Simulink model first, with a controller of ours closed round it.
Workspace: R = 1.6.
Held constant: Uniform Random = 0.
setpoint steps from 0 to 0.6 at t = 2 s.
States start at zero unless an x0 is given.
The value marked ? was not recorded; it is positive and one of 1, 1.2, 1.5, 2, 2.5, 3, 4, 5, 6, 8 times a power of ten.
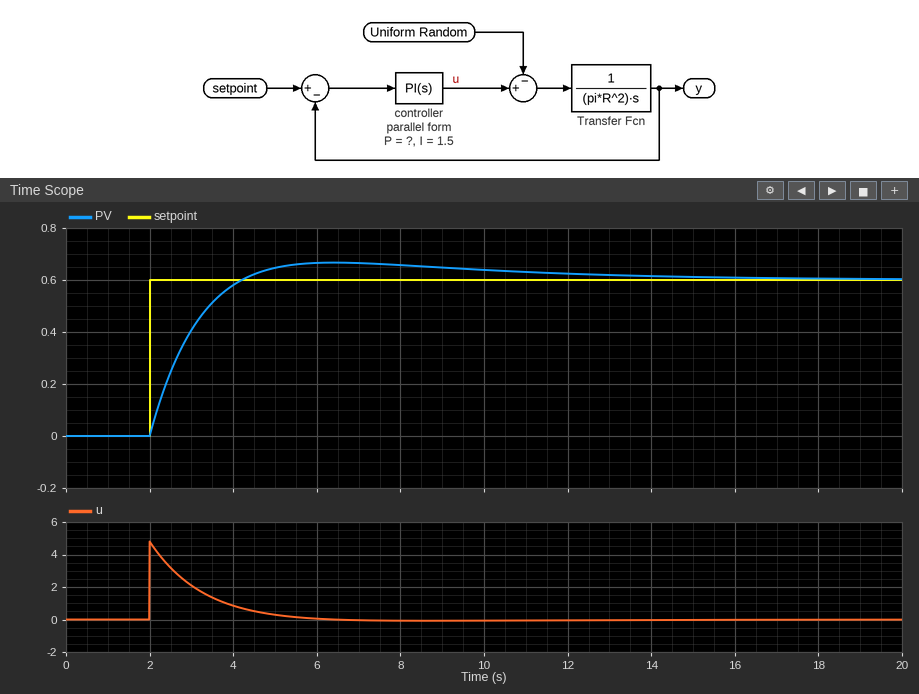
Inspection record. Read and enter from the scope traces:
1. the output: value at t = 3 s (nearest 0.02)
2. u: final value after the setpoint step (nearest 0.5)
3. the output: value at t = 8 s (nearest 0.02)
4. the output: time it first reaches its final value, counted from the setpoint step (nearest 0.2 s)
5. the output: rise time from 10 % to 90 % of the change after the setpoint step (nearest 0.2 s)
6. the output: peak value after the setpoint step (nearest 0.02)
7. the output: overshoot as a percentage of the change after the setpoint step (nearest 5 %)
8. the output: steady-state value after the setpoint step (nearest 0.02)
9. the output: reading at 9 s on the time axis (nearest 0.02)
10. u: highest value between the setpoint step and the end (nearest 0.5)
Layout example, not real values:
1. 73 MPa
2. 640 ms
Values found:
1. 0.40
2. 0.0
3. 0.66
4. 2.2 s
5. 1.6 s
6. 0.66
7. 10 %
8. 0.60
9. 0.64
10. 5.0
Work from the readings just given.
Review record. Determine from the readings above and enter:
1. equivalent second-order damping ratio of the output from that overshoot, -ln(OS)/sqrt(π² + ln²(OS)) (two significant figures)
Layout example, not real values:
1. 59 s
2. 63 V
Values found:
1. 0.59
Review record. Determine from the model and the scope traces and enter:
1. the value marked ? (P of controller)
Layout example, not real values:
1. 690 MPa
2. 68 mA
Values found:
1. 8
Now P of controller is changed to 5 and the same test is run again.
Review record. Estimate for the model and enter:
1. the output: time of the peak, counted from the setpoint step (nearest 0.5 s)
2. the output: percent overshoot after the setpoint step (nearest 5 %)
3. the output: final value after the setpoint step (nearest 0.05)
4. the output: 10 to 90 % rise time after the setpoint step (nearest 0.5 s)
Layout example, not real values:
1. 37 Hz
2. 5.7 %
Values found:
1. 5.0 s
2. 20 %
3. 0.60
4. 2.0 s
